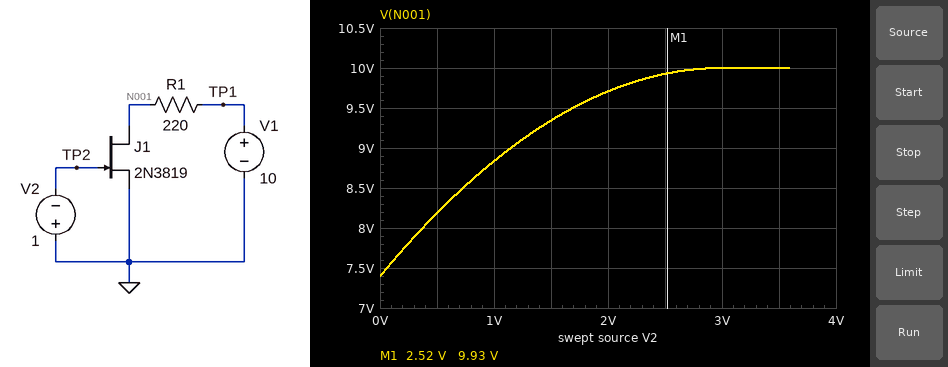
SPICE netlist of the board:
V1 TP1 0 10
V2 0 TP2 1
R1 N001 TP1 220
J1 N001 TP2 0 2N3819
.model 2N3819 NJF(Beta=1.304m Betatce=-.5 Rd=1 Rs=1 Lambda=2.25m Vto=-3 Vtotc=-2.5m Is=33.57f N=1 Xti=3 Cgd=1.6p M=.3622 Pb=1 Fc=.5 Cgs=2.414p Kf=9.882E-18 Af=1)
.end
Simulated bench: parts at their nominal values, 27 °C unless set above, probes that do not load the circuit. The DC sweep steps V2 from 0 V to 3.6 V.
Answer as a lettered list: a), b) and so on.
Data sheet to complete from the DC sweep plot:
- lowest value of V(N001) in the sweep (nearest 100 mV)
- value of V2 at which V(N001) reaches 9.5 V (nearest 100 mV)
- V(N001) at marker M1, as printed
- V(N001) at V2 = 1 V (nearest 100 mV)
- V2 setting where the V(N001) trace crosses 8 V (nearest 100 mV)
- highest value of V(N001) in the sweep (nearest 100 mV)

a) 7.4 V
b) 1.7 V
c) 9.93 V
d) 8.8 V
e) 400 mV
f) 10.0 V
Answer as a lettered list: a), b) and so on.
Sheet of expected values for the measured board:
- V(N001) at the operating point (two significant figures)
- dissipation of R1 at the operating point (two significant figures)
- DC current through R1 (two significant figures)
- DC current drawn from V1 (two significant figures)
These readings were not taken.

a) 8.8 V
b) 6.2 mW
c) 5.3 mA
d) 5.3 mA
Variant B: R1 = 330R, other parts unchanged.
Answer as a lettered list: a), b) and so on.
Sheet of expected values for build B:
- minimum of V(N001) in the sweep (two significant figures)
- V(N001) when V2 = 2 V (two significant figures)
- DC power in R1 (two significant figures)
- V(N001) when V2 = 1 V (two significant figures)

a) 6.1 V
b) 9.6 V
c) 9.2 mW
d) 8.3 V
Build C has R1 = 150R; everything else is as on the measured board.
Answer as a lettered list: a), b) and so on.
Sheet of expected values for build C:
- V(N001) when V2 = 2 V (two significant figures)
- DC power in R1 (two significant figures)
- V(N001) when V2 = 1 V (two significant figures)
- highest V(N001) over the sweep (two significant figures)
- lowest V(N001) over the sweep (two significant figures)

a) 9.8 V
b) 4.2 mW
c) 9.2 V
d) 10 V
e) 8.2 V
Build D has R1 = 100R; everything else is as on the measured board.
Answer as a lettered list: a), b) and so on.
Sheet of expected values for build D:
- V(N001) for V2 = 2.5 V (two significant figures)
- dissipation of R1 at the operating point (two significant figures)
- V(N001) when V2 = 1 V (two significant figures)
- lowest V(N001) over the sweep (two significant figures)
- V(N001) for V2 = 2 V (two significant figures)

a) 10 V
b) 2.8 mW
c) 9.5 V
d) 8.8 V
e) 9.9 V
